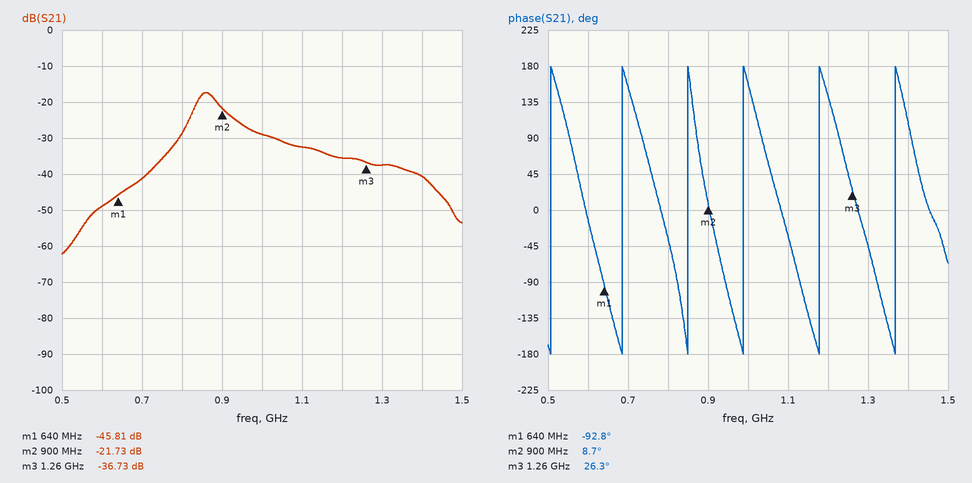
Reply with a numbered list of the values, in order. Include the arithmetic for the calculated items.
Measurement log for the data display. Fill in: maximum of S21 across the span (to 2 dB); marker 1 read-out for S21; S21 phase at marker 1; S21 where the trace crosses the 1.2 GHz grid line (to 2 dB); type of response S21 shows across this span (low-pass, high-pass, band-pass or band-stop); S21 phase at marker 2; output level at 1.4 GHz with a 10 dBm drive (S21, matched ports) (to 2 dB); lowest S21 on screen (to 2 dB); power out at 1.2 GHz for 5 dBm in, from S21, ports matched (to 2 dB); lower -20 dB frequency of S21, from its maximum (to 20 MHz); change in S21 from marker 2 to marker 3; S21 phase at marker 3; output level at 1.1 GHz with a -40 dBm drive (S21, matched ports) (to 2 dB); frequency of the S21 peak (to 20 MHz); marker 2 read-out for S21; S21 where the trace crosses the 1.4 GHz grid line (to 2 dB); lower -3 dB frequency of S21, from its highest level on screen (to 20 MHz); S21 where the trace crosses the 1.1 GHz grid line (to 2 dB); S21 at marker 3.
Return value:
1. -18 dB
2. -45.81 dB
3. -92.8°
4. -36 dB
5. band-pass
6. 8.7°
7. 10 dBm + (-40 dB) = -30 dBm
8. -62 dB
9. 5 dBm + (-36 dB) = -30 dBm
10. 740 MHz
11. -36.73 − (-21.73) = -15.00 dB
12. 26.3°
13. -40 dBm + (-32 dB) = -72 dBm
14. 860 MHz
15. -21.73 dB
16. -40 dB
17. 840 MHz
18. -32 dB
19. -36.73 dB
